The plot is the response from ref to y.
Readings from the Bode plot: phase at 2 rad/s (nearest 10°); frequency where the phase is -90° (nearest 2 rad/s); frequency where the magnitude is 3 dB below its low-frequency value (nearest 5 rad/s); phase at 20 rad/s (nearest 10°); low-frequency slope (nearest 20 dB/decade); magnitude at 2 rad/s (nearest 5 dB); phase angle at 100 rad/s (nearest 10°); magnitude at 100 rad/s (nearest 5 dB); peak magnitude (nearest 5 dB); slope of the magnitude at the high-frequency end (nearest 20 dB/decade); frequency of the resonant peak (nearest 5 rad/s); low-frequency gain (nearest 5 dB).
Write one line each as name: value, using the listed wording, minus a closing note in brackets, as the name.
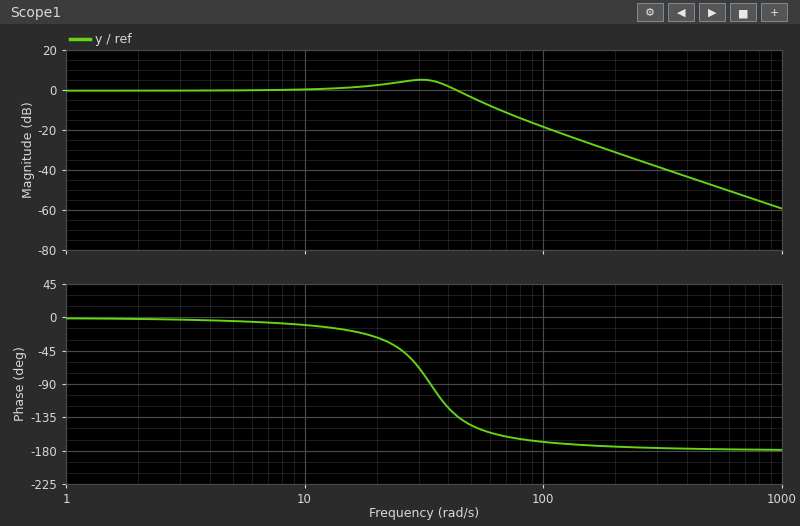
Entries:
phase at 2 rad/s: 0°
frequency where the phase is -90°: 34 rad/s
frequency where the magnitude is 3 dB below its low-frequency value: 50 rad/s
phase at 20 rad/s: -30°
low-frequency slope: 0 dB/decade
magnitude at 2 rad/s: 0 dB
phase angle at 100 rad/s: -170°
magnitude at 100 rad/s: -20 dB
peak magnitude: 5 dB
slope of the magnitude at the high-frequency end: -40 dB/decade
frequency of the resonant peak: 30 rad/s
low-frequency gain: 0 dB
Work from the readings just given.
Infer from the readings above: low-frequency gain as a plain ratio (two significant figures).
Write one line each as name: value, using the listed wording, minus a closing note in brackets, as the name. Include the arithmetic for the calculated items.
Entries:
low-frequency gain as a plain ratio: 10^(0 / 20) = 1.0
